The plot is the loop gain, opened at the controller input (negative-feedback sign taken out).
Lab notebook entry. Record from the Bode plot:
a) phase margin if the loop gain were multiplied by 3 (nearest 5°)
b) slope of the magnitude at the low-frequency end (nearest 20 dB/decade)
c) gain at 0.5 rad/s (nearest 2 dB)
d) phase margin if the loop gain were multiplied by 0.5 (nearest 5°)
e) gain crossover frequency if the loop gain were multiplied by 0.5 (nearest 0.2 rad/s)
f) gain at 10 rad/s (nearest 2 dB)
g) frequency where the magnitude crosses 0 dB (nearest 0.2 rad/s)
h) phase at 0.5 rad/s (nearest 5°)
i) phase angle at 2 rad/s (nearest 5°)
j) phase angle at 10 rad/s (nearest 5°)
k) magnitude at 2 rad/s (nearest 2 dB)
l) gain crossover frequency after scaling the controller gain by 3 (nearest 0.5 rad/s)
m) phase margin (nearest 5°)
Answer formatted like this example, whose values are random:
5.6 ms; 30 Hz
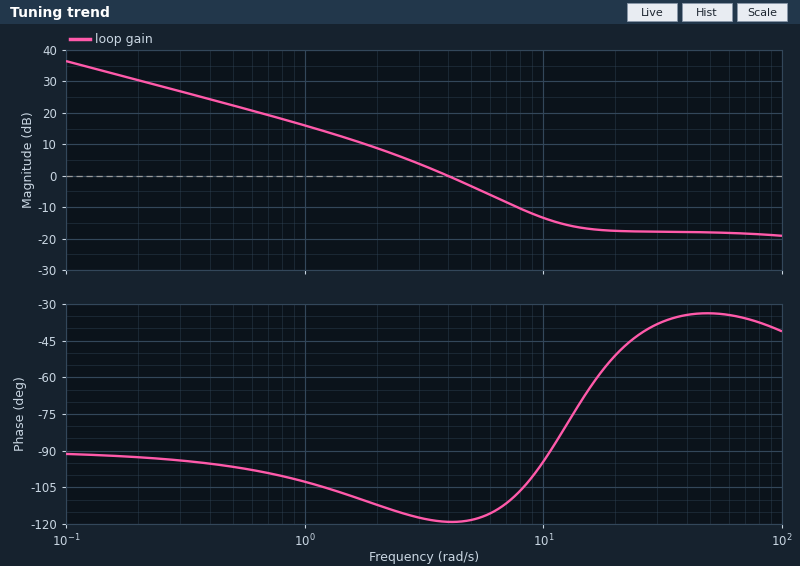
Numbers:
70°; -20 dB/decade; 22 dB; 65°; 2.6 rad/s; -14 dB; 4.0 rad/s; -95°; -110°; -95°; 8 dB; 7.5 rad/s; 60°
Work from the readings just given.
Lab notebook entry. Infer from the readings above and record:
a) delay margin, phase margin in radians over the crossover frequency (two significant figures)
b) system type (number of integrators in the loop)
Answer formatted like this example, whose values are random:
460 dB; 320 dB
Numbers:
0.26 s; 1
